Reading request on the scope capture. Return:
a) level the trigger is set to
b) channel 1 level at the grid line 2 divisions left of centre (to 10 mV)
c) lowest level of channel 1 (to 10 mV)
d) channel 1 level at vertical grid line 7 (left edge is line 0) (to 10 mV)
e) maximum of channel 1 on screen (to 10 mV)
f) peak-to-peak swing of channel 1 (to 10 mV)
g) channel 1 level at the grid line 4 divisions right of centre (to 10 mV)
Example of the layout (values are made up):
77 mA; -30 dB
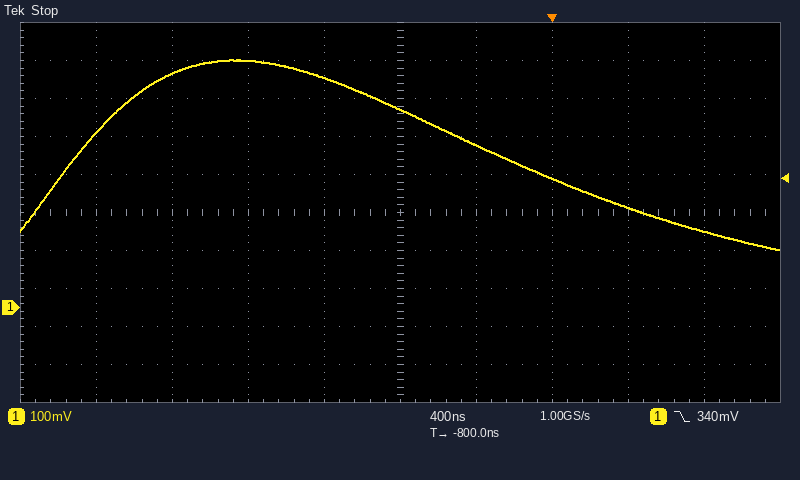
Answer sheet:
340 mV; 650 mV; 150 mV; 340 mV; 650 mV; 500 mV; 200 mV
